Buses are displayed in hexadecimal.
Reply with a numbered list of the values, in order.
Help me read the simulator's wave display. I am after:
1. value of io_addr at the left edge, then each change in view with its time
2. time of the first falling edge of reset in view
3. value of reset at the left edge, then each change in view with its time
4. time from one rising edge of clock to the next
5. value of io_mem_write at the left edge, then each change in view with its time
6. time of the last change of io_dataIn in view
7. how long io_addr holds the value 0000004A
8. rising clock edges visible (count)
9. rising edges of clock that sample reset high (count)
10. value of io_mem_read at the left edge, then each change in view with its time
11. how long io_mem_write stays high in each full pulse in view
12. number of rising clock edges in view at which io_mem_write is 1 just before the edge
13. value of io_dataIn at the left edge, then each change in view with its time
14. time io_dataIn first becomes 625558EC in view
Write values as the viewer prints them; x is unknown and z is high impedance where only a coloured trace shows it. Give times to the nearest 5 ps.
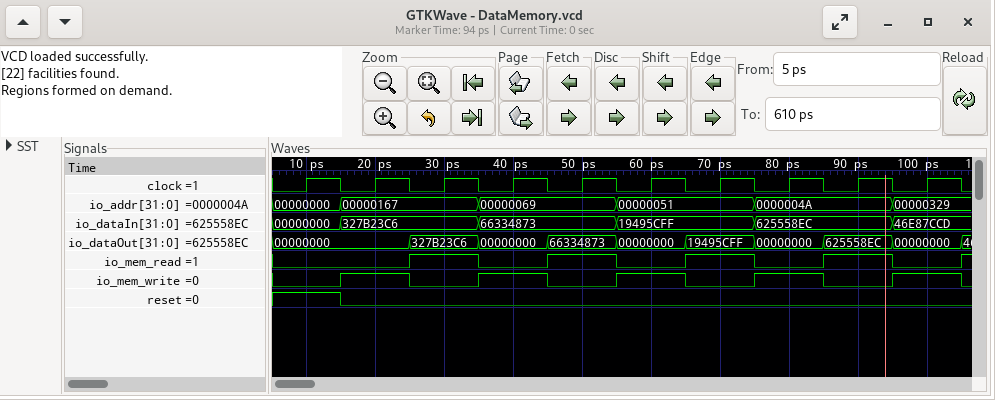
1. 00000000, 00000167 at 15 ps, 00000069 at 35 ps, 00000051 at 55 ps, 0000004A at 75 ps, 00000329 at 95 ps
2. 15 ps
3. 1, 0 at 15 ps
4. 10 ps
5. 0, 1 at 15 ps, 0 at 25 ps, 1 at 35 ps, 0 at 45 ps, 1 at 55 ps, 0 at 65 ps, 1 at 75 ps, 0 at 85 ps, 1 at 95 ps, 0 at 105 ps
6. 95 ps
7. 20 ps
8. 10
9. 1
10. 0, 1 at 25 ps, 0 at 35 ps, 1 at 45 ps, 0 at 55 ps, 1 at 65 ps, 0 at 75 ps, 1 at 85 ps, 0 at 95 ps, 1 at 105 ps
11. 10 ps, 10 ps, 10 ps, 10 ps, 10 ps
12. 5
13. 00000000, 327B23C6 at 15 ps, 66334873 at 35 ps, 19495CFF at 55 ps, 625558EC at 75 ps, 46E87CCD at 95 ps
14. 75 ps
